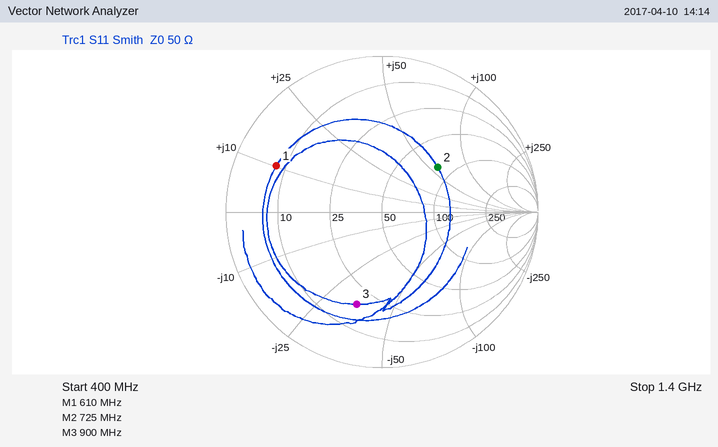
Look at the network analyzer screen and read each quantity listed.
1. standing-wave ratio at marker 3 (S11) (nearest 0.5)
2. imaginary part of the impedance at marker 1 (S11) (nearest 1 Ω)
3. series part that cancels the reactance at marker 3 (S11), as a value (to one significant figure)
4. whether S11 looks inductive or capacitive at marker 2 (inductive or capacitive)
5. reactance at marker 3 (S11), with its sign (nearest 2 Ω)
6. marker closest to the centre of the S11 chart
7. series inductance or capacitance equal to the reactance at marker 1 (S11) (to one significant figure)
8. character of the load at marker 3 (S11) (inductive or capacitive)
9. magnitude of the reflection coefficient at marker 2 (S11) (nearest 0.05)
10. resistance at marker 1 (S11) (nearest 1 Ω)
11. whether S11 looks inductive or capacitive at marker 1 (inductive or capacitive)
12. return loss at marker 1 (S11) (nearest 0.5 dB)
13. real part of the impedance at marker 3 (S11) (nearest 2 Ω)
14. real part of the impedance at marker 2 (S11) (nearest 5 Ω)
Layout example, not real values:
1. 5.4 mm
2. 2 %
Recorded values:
1. 4.0
2. +10 Ω
3. 6 nH
4. inductive
5. -34 Ω
6. marker 2
7. 3 nH
8. capacitive
9. 0.45
10. 8 Ω
11. inductive
12. 2.5 dB
13. 18 Ω
14. 80 Ω
